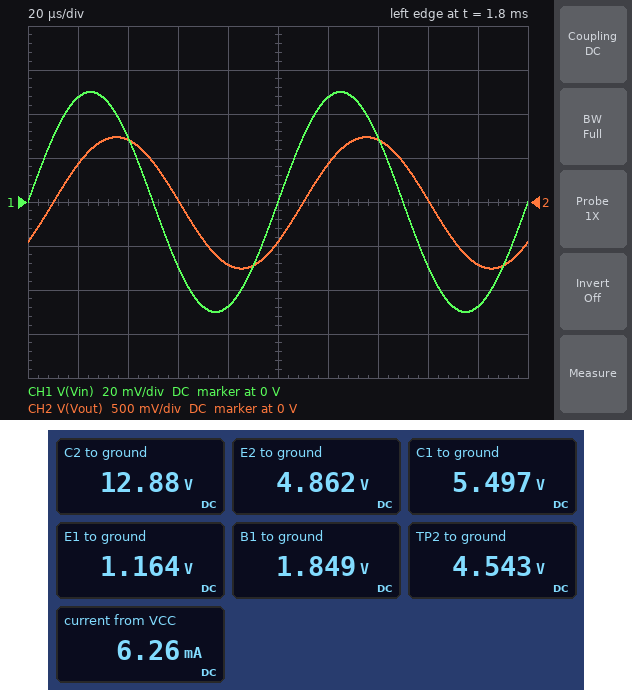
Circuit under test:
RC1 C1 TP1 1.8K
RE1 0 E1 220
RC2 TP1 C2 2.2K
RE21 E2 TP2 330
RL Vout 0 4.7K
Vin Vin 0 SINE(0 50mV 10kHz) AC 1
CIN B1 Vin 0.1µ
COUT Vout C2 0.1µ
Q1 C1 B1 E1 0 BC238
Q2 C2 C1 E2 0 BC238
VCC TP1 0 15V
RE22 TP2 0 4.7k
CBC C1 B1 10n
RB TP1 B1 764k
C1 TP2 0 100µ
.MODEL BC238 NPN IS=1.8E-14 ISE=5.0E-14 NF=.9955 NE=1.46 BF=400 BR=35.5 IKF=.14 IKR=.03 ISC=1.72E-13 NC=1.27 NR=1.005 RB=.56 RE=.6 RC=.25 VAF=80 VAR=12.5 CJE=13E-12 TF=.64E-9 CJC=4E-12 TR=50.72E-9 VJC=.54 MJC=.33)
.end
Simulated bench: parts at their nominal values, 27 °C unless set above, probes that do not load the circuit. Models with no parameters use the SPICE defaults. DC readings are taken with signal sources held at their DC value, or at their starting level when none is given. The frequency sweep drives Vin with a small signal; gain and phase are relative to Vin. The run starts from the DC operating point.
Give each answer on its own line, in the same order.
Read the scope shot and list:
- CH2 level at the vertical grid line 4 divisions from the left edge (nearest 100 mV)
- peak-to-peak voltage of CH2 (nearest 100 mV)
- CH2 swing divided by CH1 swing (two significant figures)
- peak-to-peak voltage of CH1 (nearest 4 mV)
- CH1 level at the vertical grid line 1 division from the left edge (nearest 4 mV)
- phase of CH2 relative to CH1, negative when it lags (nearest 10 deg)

-700 mV
1.5 V
15
100 mV
48 mV
-40 deg
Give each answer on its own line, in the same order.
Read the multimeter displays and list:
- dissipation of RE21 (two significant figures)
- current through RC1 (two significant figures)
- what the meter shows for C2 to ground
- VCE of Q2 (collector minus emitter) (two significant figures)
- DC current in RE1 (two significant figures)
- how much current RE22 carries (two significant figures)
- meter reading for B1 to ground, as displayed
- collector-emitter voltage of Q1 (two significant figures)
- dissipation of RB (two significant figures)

310 µW
5.3 mA
12.88 V
8.0 V
5.3 mA
970 µA
1.849 V
4.3 V
230 µW
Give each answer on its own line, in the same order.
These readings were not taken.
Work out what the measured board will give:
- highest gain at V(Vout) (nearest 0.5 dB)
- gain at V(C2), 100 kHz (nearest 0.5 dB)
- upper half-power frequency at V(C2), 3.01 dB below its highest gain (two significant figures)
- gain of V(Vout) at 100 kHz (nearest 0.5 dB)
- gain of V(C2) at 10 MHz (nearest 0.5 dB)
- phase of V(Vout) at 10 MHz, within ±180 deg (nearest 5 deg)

24.5 dB
14.0 dB
2.9 kHz
14.0 dB
12.5 dB
165 deg
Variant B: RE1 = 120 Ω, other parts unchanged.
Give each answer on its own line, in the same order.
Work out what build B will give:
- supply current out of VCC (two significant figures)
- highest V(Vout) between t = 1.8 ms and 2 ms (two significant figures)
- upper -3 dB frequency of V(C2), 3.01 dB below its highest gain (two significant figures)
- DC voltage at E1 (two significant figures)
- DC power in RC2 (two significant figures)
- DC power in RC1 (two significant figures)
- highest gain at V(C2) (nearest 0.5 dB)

6.4 mA
1.0 V
5.0 kHz
660 mV
1.7 mW
54 mW
30.0 dB
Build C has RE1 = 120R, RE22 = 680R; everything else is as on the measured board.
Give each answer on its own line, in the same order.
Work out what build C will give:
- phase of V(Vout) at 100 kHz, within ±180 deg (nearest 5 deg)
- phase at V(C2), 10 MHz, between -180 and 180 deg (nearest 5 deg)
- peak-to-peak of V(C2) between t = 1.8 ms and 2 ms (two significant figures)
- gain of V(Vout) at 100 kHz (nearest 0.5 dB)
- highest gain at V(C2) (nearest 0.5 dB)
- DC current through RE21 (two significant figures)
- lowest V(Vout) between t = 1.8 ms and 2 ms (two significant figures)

-115 deg
155 deg
1.9 V
17.0 dB
30.5 dB
4.4 mA
-870 mV
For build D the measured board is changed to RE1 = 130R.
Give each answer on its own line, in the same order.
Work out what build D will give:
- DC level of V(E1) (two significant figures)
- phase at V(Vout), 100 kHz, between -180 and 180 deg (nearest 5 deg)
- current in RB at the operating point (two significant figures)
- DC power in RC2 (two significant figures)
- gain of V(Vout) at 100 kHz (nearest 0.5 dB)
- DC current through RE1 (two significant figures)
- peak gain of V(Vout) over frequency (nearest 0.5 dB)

710 mV
-120 deg
18 µA
1.8 mW
16.0 dB
5.5 mA
27.0 dB
